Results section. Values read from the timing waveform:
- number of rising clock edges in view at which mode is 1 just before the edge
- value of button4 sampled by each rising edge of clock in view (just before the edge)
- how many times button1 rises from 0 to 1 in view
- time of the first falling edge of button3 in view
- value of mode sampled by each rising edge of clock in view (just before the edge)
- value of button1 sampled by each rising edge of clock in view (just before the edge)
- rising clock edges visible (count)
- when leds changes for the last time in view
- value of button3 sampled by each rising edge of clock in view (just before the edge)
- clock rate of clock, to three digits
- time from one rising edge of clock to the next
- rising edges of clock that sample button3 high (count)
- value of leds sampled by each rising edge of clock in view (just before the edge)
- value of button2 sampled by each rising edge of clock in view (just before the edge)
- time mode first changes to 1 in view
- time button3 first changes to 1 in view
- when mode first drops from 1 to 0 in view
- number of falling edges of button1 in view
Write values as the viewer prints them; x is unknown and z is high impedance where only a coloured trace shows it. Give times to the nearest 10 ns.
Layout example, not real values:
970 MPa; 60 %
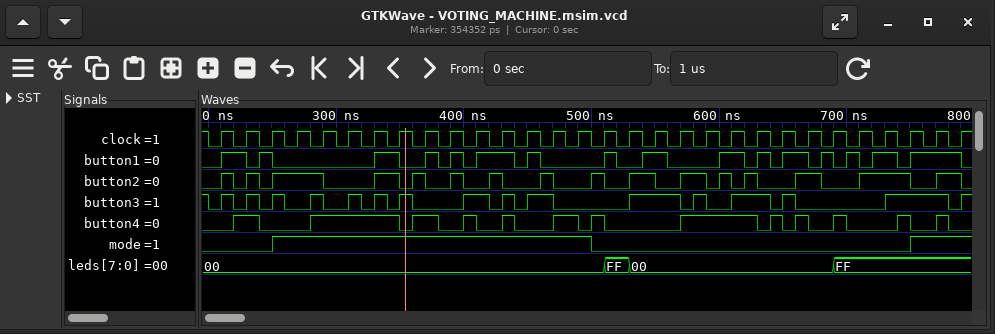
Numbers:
14; 0 1 0 0 1 1 1 1 1 0 1 0 0 0 1 1 0 0 0 1 1 1 1 1 0 0 0 1 0 0; 16; 200 ns; 0 0 0 1 1 1 1 1 1 1 1 1 1 1 1 0 0 0 0 0 0 0 0 0 0 0 0 0 1 1; 0 1 1 0 0 0 0 1 0 0 0 1 0 0 0 0 0 1 0 0 1 0 0 1 1 1 1 0 1 1; 30; 690 ns; 0 0 0 0 1 0 0 0 0 0 1 0 0 1 0 0 0 1 1 1 0 1 0 0 0 0 0 1 1 0; 50.0 MHz; 20 ns; 9; 00, 00, 00, 00, 00, 00, 00, 00, 00, 00, 00, 00, 00, 00, 00, 00, FF, 00, 00, 00, 00, 00, 00, 00, 00, FF, FF, FF, FF, FF; 0 0 0 1 1 0 0 1 1 0 0 1 0 1 0 1 0 1 0 1 1 1 0 1 0 0 1 1 0 1; 250 ns; 210 ns; 500 ns; 16
